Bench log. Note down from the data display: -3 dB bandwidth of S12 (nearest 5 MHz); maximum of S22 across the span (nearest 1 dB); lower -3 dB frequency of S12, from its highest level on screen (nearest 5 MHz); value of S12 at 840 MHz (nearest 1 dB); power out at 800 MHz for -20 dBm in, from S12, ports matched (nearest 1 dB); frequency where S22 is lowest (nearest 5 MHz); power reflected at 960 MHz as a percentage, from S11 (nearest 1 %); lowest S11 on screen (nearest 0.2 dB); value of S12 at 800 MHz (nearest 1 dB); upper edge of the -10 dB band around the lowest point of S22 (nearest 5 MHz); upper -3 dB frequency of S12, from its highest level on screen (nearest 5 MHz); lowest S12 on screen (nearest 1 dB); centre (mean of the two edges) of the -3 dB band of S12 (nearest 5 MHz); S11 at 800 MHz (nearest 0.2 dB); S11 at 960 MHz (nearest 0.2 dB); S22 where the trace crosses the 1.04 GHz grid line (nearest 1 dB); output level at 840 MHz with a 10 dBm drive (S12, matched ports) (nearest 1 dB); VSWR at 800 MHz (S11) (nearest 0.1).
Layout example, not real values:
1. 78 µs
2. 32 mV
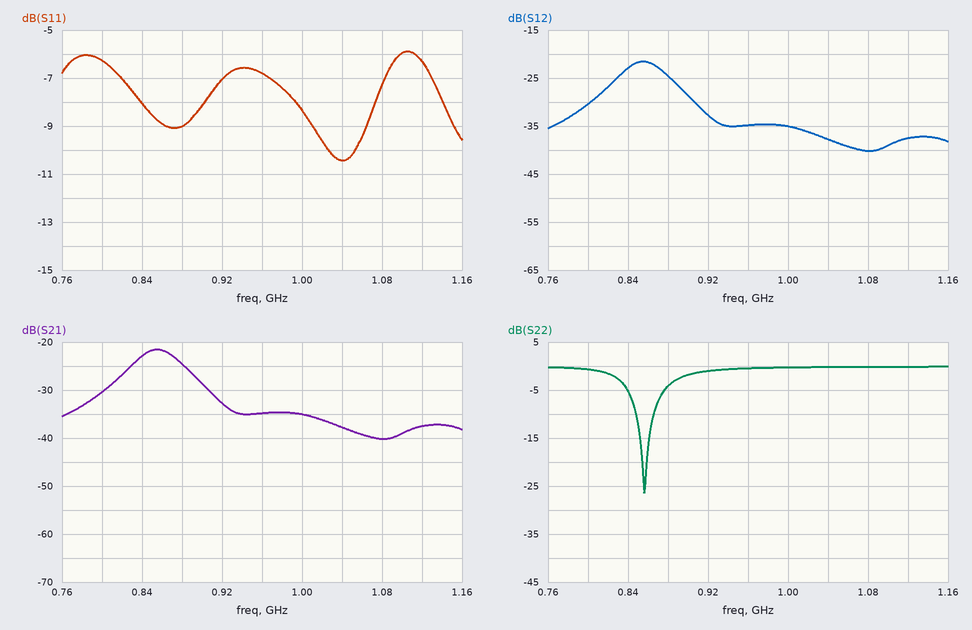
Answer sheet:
1. 50 MHz
2. 0 dB
3. 830 MHz
4. -23 dB
5. -50 dBm
6. 855 MHz
7. 21 %
8. -10.4 dB
9. -30 dB
10. 865 MHz
11. 880 MHz
12. -40 dB
13. 855 MHz
14. -6.2 dB
15. -6.8 dB
16. 0 dB
17. -13 dBm
18. 2.9
